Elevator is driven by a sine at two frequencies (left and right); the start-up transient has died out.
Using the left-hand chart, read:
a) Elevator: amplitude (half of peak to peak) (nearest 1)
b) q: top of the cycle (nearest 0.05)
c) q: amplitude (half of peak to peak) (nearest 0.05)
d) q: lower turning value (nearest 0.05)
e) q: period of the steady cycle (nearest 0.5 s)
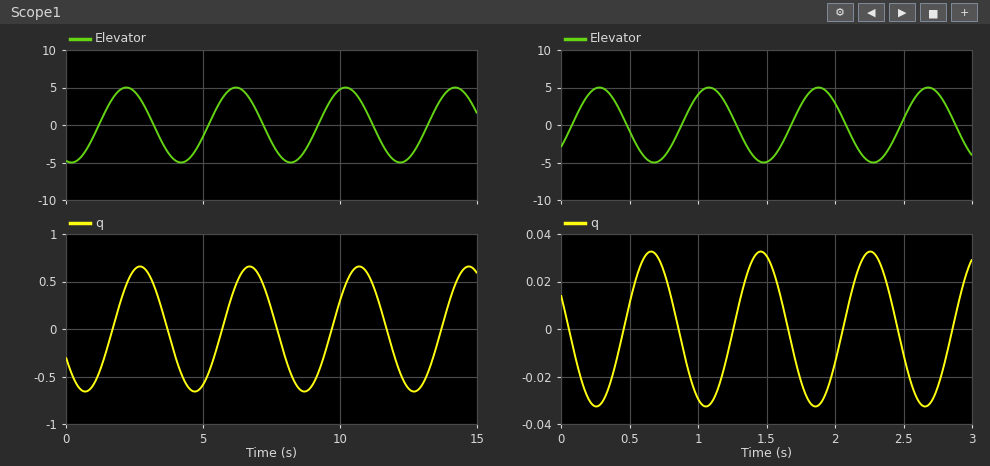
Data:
5
0.65
0.65
-0.65
4.0 s
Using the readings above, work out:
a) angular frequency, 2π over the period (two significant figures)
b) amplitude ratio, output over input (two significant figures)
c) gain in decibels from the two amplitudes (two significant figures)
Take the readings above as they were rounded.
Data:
1.6 rad/s
0.13
-18 dB
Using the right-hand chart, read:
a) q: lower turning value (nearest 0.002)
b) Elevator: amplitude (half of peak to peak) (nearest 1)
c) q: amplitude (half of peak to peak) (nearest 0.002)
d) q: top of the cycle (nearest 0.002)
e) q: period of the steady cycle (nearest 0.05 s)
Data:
-0.032
5
0.032
0.032
0.80 s
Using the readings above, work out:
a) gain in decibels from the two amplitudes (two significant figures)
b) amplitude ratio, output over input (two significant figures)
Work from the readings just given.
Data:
-44 dB
0.0064
